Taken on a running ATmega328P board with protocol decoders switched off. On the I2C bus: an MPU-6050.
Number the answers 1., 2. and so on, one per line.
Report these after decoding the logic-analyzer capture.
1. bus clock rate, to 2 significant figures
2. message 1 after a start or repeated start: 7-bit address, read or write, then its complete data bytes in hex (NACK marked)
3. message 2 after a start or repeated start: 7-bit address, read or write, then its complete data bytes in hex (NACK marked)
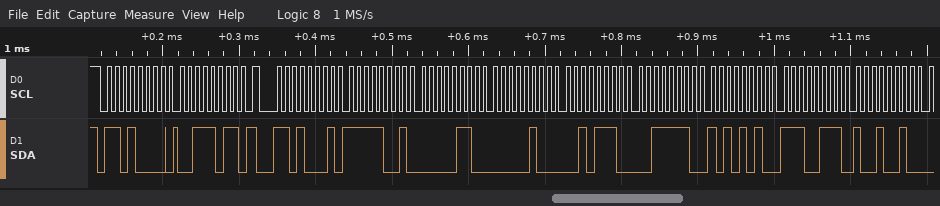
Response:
1. 100 kHz
2. 0x68 write: 3B
3. 0x68 read: F9 06 04 2E 3E AA E7 92
